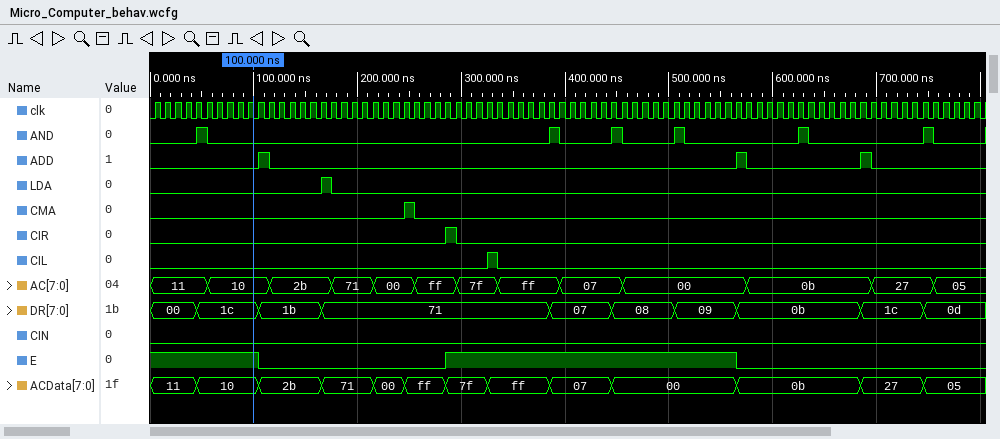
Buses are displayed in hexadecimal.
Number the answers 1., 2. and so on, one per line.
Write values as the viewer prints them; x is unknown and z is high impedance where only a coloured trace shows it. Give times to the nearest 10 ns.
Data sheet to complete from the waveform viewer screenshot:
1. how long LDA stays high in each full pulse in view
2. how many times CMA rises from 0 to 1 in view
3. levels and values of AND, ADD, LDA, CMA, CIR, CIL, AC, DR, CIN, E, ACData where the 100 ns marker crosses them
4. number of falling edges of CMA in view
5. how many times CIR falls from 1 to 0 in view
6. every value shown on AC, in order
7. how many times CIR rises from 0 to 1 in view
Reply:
1. 10 ns
2. 1
3. AND=0, ADD=0, LDA=0, CMA=0, CIR=0, CIL=0, AC=10, DR=1c, CIN=0, E=1, ACData=10
4. 1
5. 1
6. 11, 10, 2b, 71, 00, ff, 7f, ff, 07, 00, 0b, 27, 05
7. 1
